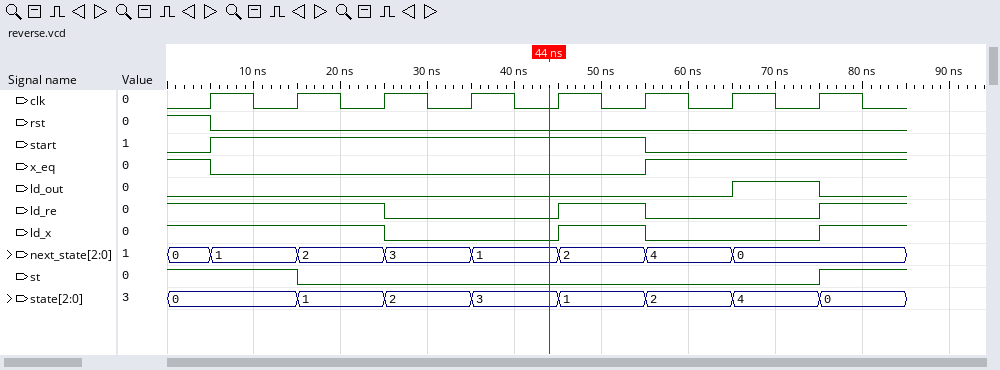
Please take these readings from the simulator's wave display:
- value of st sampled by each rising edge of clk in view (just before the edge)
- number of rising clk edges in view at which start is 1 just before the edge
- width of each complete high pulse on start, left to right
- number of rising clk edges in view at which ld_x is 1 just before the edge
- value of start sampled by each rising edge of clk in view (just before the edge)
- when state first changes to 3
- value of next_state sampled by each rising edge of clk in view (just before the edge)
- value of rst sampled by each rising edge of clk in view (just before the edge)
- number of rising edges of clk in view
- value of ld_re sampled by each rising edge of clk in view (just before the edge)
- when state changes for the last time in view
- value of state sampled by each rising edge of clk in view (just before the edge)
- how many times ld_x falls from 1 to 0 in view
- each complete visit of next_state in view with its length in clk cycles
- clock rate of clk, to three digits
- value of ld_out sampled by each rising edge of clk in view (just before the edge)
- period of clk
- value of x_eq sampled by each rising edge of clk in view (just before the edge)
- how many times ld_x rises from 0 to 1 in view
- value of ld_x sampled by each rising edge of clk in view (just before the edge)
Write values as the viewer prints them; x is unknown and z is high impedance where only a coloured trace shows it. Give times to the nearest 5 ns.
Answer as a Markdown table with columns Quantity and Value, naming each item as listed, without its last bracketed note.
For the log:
| Quantity | Value |
|---|---|
| value of st sampled by each rising edge of clk in view | 1 1 0 0 0 0 0 0 |
| number of rising clk edges in view at which start is 1 just before the edge | 5 |
| width of each complete high pulse on start, left to right | 50 ns |
| number of rising clk edges in view at which ld_x is 1 just before the edge | 4 |
| value of start sampled by each rising edge of clk in view | 0 1 1 1 1 1 0 0 |
| when state first changes to 3 | 35 ns |
| value of next_state sampled by each rising edge of clk in view | 0, 1, 2, 3, 1, 2, 4, 0 |
| value of rst sampled by each rising edge of clk in view | 1 0 0 0 0 0 0 0 |
| number of rising edges of clk in view | 8 |
| value of ld_re sampled by each rising edge of clk in view | 1 1 1 0 0 1 0 0 |
| when state changes for the last time in view | 75 ns |
| value of state sampled by each rising edge of clk in view | 0, 0, 1, 2, 3, 1, 2, 4 |
| how many times ld_x falls from 1 to 0 in view | 2 |
| each complete visit of next_state in view with its length in clk cycles | 1: 1, 2: 1, 3: 1, 1: 1, 2: 1, 4: 1 |
| clock rate of clk, to three digits | 100 MHz |
| value of ld_out sampled by each rising edge of clk in view | 0 0 0 0 0 0 0 1 |
| period of clk | 10 ns |
| value of x_eq sampled by each rising edge of clk in view | 1 0 0 0 0 0 1 1 |
| how many times ld_x rises from 0 to 1 in view | 2 |
| value of ld_x sampled by each rising edge of clk in view | 1 1 1 0 0 1 0 0 |
